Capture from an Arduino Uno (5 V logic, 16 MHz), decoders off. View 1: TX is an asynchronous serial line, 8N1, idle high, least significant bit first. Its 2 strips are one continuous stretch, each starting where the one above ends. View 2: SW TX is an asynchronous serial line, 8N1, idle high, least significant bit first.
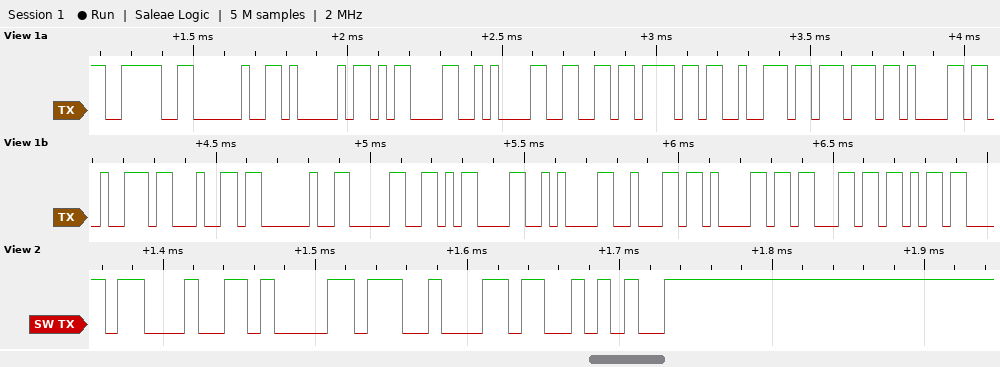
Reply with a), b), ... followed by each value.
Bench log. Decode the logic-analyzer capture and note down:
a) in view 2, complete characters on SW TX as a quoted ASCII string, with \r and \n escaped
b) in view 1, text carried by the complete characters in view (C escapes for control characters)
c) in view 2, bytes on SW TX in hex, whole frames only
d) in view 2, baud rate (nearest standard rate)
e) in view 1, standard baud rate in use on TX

a) "#ab*"
b) "> A\r\nforward 0\r\nback"
c) 0x23 0x61 0x62 0x2A
d) 115200 baud
e) 38400 baud
